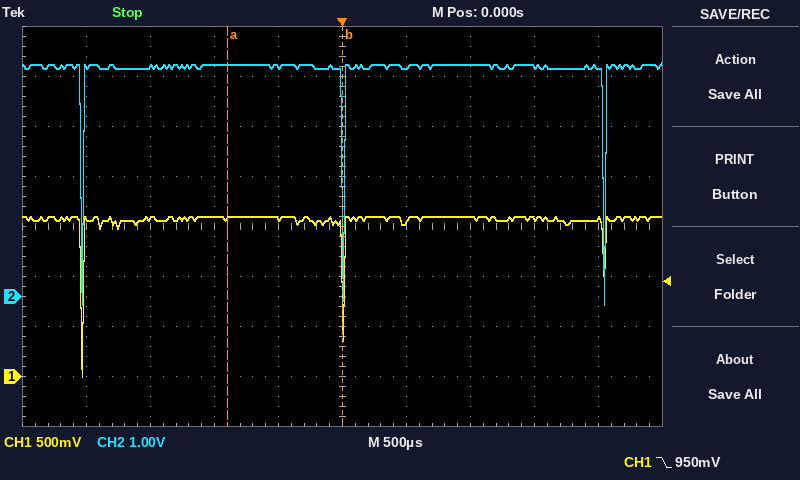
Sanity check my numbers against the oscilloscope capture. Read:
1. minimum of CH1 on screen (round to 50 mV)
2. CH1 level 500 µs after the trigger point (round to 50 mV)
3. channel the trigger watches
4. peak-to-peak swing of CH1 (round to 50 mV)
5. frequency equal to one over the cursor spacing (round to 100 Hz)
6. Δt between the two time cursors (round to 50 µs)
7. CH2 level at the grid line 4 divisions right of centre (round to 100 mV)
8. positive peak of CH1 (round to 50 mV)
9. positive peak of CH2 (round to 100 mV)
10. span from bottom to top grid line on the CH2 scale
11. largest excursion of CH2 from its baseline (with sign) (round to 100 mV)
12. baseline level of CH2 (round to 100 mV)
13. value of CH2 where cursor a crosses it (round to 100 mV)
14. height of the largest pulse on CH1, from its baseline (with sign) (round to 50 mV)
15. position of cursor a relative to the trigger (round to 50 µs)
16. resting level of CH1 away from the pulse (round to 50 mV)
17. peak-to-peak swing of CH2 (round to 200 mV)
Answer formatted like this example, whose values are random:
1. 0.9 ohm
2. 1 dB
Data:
1. 0 mV
2. 1.55 V
3. CH1
4. 1.60 V
5. 1.1 kHz
6. 900 µs
7. 4.6 V
8. 1.60 V
9. 4.7 V
10. 8 V
11. -4.8 V
12. 4.6 V
13. 4.6 V
14. -1.60 V
15. -900 µs
16. 1.60 V
17. 4.8 V
